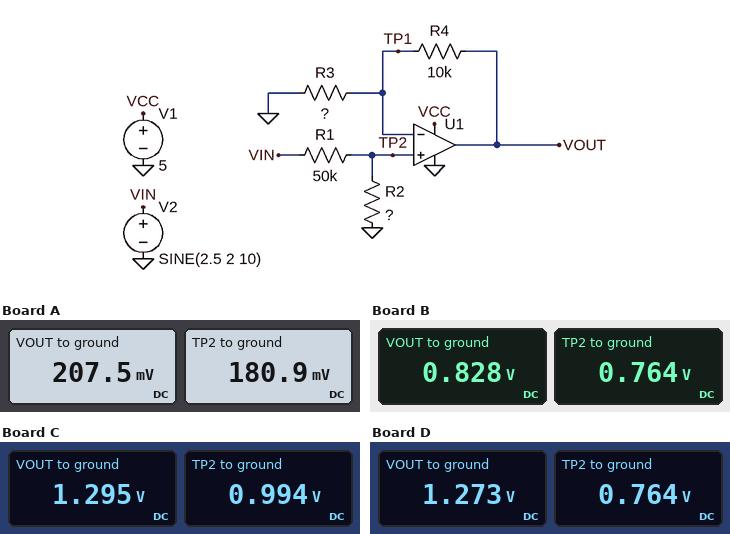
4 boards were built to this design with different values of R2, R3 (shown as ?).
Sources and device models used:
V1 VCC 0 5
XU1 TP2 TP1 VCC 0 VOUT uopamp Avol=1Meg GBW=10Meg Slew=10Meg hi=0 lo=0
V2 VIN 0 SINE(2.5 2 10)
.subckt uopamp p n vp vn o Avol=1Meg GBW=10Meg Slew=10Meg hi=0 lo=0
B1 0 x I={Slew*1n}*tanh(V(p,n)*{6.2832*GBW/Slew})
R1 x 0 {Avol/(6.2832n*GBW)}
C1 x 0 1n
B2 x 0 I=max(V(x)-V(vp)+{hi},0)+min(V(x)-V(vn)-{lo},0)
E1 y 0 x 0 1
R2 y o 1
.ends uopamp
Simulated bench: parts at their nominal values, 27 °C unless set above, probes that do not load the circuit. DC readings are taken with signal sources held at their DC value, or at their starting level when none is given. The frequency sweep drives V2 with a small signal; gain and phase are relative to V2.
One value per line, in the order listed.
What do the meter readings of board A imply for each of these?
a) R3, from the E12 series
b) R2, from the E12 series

68 kΩ
3.9 kΩ
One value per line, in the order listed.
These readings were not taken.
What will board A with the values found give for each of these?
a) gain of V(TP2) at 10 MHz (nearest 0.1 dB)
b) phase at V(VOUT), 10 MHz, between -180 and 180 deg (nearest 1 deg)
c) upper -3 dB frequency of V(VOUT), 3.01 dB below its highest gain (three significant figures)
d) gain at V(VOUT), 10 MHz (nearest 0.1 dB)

-22.8 dB
-49 deg
8.72 MHz
-25.3 dB
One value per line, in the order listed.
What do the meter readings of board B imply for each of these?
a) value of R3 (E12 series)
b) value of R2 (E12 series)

120 kΩ
22 kΩ
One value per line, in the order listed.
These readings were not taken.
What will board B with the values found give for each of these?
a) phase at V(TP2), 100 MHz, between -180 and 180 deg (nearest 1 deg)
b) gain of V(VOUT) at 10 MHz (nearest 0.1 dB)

0 deg
-13.0 dB
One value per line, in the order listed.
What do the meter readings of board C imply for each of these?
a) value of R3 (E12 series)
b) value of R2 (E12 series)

33 kΩ
33 kΩ
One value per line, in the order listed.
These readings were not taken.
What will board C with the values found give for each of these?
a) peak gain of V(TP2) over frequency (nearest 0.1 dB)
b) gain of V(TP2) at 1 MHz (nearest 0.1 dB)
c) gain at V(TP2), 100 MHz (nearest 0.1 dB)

-8.0 dB
-8.0 dB
-8.0 dB
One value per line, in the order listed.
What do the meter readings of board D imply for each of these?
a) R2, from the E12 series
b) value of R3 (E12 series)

22 kΩ
15 kΩ
